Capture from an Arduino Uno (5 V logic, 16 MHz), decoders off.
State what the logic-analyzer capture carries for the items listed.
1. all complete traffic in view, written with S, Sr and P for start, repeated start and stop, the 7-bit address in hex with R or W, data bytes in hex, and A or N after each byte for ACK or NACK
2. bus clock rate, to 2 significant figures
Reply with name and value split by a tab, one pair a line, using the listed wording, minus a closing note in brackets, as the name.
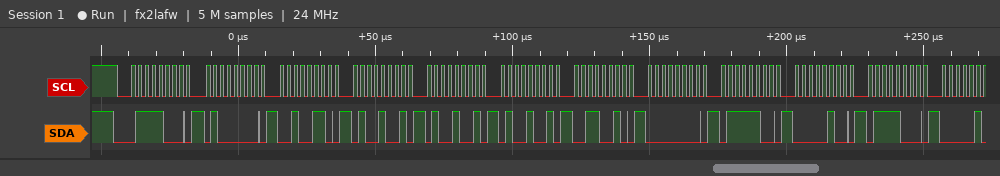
all complete traffic in view, written with S, Sr and P for start, repeated start and stop, the 7-bit address in hex with R or W, data bytes in hex, and A or N after each byte for ACK or NACK	S 3CW A 40 A 26 A 49 A 49 A 49 A 32 A 00 A 7C A 04 A 78 A
bus clock rate, to 2 significant figures	400 kHz
